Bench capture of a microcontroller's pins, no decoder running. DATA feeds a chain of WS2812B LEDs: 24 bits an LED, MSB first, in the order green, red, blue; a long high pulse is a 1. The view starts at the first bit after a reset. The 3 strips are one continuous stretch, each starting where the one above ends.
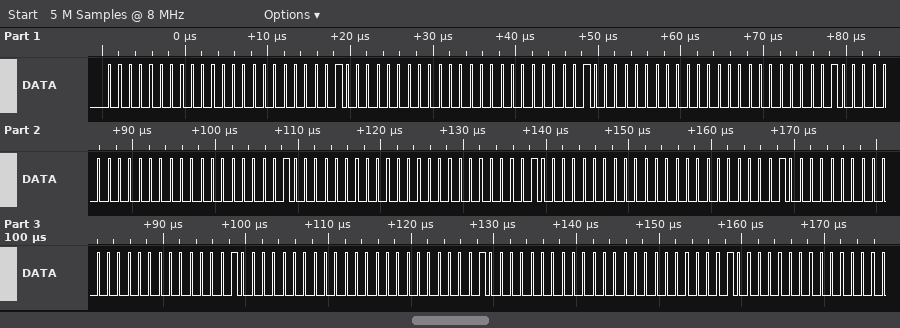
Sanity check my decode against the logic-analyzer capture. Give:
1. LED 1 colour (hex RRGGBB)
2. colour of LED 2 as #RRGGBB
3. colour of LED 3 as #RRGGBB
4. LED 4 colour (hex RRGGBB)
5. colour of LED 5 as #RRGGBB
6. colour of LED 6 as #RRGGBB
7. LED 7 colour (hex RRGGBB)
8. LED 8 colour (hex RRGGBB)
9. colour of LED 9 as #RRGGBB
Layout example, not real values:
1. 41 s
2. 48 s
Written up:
1. #000002
2. #000002
3. #000002
4. #000002
5. #000002
6. #000002
7. #000002
8. #000002
9. #000002
